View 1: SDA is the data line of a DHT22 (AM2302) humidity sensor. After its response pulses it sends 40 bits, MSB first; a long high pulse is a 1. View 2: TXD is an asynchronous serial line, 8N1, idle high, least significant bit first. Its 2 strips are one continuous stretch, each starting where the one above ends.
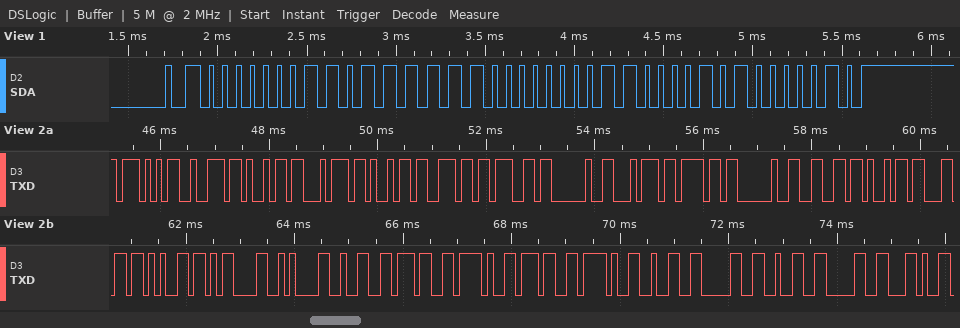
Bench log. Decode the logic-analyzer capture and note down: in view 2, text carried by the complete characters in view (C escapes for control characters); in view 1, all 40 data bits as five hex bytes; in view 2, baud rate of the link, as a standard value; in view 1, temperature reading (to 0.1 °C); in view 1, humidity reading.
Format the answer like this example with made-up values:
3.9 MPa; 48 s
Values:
"Writing to file\r\n27/7/2020,"; 01 BF 00 C2 82; 9600 baud; 19.4 °C; 44.7 %
